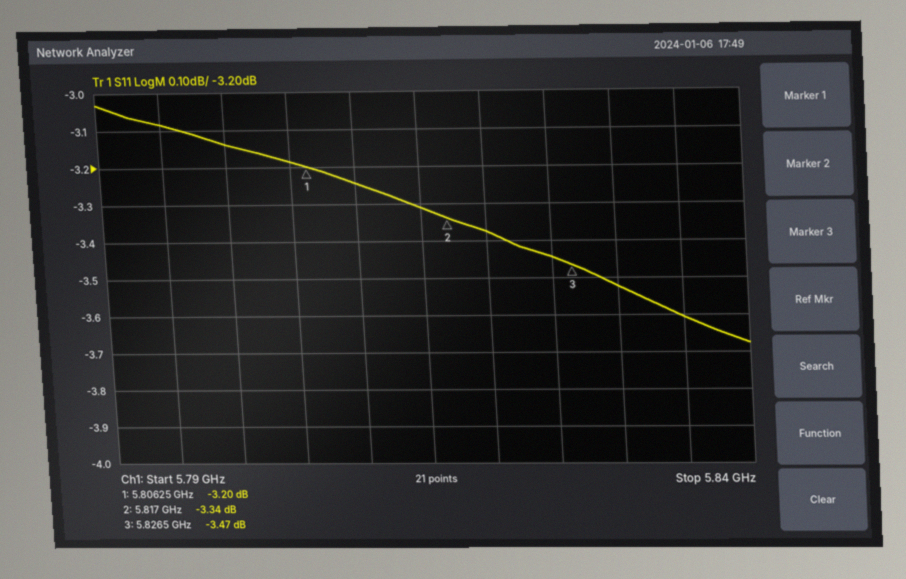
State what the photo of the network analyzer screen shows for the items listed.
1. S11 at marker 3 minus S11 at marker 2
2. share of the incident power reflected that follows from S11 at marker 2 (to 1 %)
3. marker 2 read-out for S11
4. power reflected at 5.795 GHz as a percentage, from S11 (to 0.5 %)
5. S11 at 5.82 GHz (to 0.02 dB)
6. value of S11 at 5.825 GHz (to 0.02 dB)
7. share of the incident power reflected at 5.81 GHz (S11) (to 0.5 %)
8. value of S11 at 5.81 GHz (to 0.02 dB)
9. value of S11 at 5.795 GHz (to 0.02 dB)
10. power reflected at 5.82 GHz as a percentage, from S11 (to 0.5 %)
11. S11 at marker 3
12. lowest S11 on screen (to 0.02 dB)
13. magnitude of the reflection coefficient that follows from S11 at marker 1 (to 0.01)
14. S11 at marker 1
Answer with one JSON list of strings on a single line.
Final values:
["-0.13 dB", "46 %", "-3.34 dB", "49.0 %", "-3.38 dB", "-3.44 dB", "47.5 %", "-3.24 dB", "-3.08 dB", "46.0 %", "-3.47 dB", "-3.68 dB", "0.69", "-3.20 dB"]
